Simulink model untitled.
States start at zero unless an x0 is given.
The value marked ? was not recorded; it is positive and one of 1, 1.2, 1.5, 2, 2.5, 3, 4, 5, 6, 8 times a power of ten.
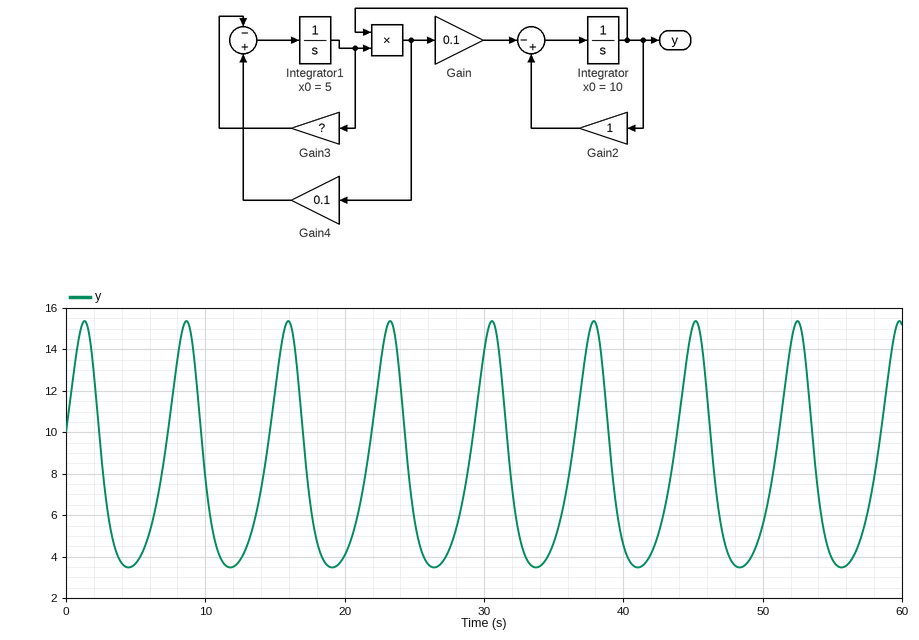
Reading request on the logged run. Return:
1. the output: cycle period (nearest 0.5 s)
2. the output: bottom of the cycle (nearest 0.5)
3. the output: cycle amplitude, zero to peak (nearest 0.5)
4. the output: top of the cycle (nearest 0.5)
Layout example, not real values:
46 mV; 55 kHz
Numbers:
7.5 s; 3.5; 6.0; 15.5
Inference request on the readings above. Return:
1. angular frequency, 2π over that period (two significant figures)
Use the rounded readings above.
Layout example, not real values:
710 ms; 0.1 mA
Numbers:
0.84 rad/s
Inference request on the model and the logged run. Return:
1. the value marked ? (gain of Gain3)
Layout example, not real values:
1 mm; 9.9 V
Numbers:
0.8
